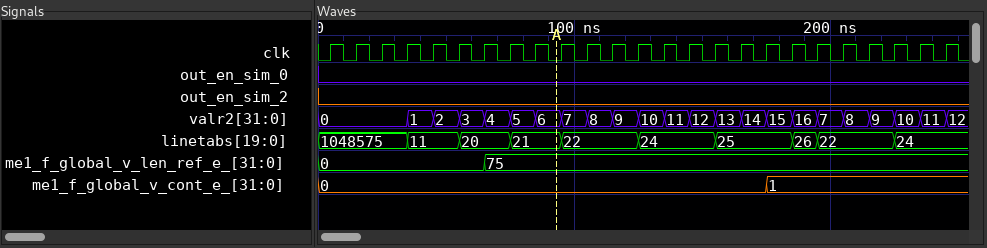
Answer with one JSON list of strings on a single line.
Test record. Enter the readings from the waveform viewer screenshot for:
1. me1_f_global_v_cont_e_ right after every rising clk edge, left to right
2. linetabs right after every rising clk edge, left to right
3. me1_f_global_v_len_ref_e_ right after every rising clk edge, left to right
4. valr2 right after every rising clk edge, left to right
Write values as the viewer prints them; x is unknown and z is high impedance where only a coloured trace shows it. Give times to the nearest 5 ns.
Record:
["0, 0, 0, 0, 0, 0, 0, 0, 0, 0, 0, 0, 0, 0, 0, 0, 0, 1, 1, 1, 1, 1, 1, 1, 1", "1048575, 1048575, 1048575, 11, 11, 20, 20, 21, 21, 22, 22, 22, 24, 24, 24, 25, 25, 25, 26, 22, 22, 22, 24, 24, 24", "0, 0, 0, 0, 0, 0, 75, 75, 75, 75, 75, 75, 75, 75, 75, 75, 75, 75, 75, 75, 75, 75, 75, 75, 75", "0, 0, 0, 1, 2, 3, 4, 5, 6, 7, 8, 9, 10, 11, 12, 13, 14, 15, 16, 7, 8, 9, 10, 11, 12"]
